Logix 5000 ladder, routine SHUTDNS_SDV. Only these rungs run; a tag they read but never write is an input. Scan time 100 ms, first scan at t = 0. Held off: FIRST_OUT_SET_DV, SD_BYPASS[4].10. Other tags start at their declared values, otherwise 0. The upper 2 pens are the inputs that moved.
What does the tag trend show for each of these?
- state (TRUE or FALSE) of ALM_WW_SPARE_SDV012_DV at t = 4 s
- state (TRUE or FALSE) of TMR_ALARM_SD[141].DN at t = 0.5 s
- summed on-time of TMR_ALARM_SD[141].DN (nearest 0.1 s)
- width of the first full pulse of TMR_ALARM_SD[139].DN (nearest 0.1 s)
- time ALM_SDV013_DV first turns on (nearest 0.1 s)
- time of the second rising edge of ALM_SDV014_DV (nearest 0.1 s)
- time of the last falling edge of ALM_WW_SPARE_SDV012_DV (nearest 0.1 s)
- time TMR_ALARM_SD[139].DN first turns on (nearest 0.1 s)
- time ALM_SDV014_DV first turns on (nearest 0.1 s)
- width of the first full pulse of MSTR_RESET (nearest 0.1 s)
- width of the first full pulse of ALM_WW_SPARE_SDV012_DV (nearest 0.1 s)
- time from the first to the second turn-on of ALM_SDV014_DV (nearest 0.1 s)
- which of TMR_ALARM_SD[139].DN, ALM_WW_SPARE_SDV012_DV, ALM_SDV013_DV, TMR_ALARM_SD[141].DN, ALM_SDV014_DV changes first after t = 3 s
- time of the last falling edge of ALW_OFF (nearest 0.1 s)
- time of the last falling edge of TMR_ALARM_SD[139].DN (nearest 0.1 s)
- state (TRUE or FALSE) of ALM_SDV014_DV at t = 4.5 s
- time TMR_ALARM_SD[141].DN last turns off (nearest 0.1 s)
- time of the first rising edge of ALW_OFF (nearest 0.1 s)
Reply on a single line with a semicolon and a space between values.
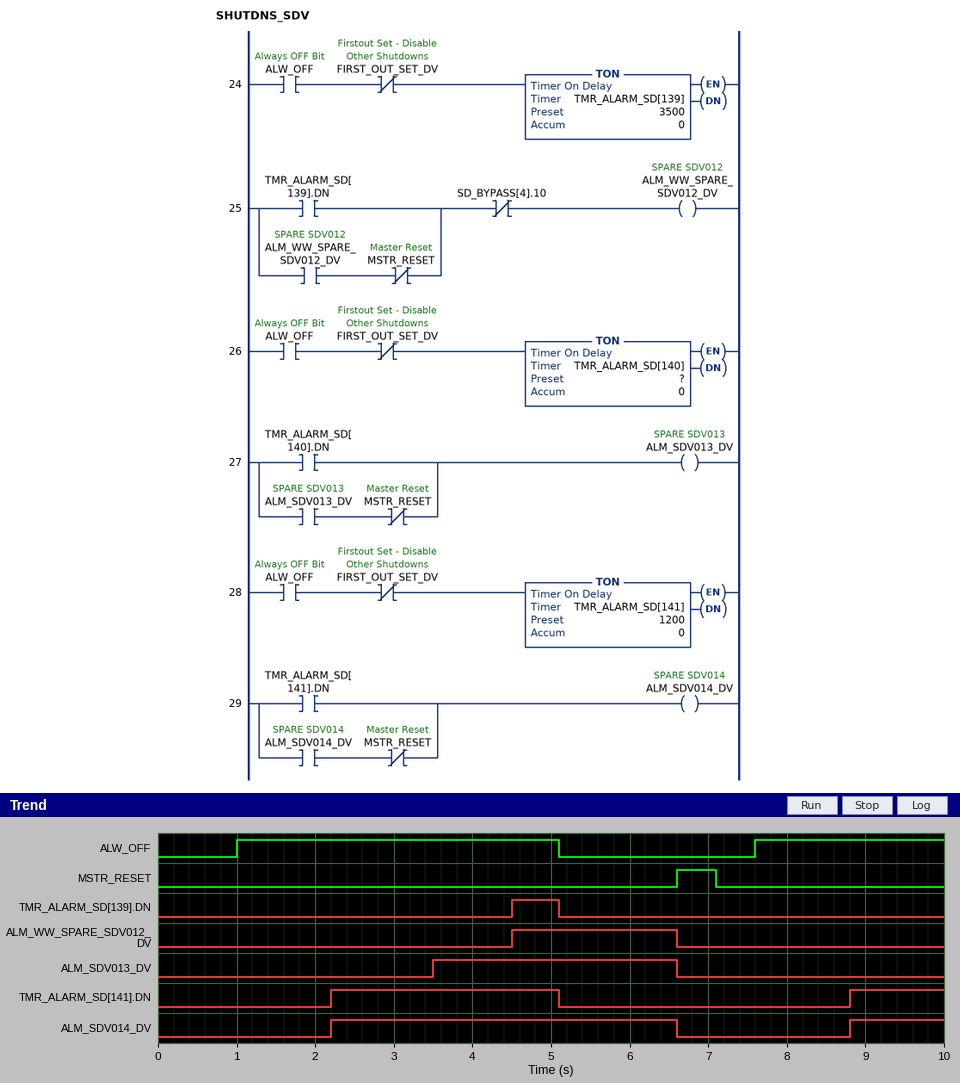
FALSE; FALSE; 4.1 s; 0.6 s; 3.5 s; 8.8 s; 6.6 s; 4.5 s; 2.2 s; 0.5 s; 2.1 s; 6.6 s; ALM_SDV013_DV; 5.1 s; 5.1 s; TRUE; 5.1 s; 1.0 s
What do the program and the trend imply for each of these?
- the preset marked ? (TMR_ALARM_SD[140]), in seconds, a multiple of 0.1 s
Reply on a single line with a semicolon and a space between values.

2.5 s
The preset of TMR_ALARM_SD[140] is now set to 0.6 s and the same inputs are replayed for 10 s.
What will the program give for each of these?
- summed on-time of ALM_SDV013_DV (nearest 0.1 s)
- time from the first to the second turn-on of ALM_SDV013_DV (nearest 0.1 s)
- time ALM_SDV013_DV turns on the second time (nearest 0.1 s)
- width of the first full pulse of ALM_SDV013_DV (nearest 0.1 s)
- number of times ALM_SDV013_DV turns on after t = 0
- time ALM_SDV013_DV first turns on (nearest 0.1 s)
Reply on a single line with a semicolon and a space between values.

6.8 s; 6.6 s; 8.2 s; 5.0 s; 2; 1.6 s
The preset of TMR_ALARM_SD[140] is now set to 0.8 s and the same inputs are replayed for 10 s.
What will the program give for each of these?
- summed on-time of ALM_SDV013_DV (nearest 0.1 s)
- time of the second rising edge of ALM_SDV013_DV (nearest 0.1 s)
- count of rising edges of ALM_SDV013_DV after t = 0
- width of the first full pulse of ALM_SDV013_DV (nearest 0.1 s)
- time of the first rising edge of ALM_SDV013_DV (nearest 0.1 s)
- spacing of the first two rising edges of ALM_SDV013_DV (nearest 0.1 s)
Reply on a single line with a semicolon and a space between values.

6.4 s; 8.4 s; 2; 4.8 s; 1.8 s; 6.6 s
